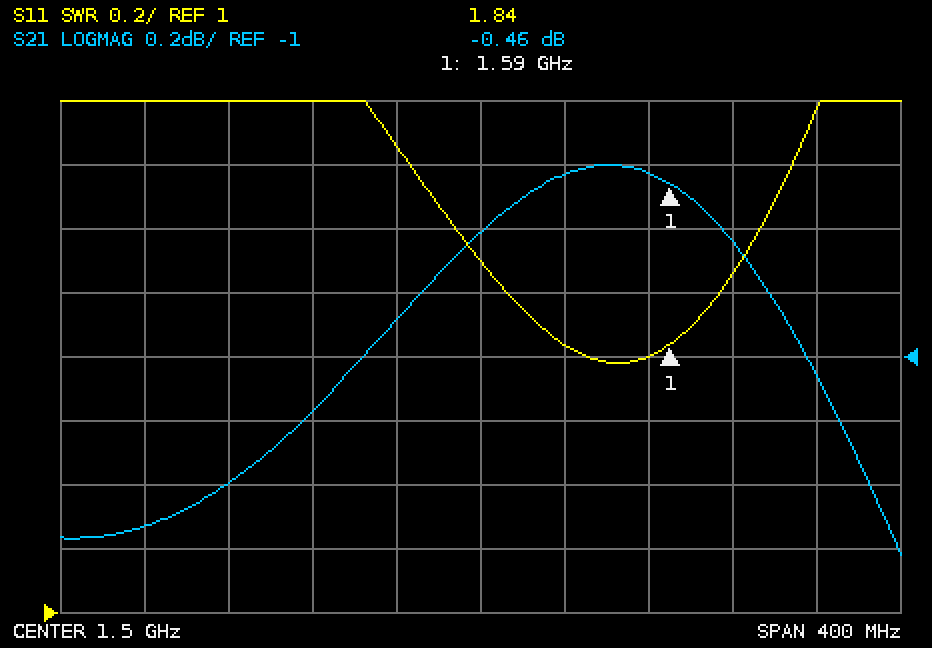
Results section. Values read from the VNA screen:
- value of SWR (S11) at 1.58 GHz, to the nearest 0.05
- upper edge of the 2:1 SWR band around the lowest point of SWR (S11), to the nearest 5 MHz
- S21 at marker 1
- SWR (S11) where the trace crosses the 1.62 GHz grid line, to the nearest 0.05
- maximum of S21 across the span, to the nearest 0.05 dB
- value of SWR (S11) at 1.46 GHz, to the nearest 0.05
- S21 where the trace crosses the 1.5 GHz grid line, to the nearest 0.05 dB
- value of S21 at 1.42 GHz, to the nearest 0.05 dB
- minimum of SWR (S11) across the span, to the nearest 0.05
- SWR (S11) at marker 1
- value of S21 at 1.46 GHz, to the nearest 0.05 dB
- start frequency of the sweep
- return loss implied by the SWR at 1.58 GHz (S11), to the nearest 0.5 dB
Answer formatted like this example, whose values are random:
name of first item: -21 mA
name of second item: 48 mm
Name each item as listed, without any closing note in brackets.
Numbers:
value of SWR (S11) at 1.58 GHz, to the nearest 0.05: 1.80
upper edge of the 2:1 SWR band around the lowest point of SWR (S11), to the nearest 5 MHz: 1.615 GHz
S21 at marker 1: -0.46 dB
SWR (S11) where the trace crosses the 1.62 GHz grid line, to the nearest 0.05: 2.05
maximum of S21 across the span, to the nearest 0.05 dB: -0.40 dB
value of SWR (S11) at 1.46 GHz, to the nearest 0.05: 2.45
S21 where the trace crosses the 1.5 GHz grid line, to the nearest 0.05 dB: -0.60 dB
value of S21 at 1.42 GHz, to the nearest 0.05 dB: -1.15 dB
minimum of SWR (S11) across the span, to the nearest 0.05: 1.80
SWR (S11) at marker 1: 1.84
value of S21 at 1.46 GHz, to the nearest 0.05 dB: -0.90 dB
start frequency of the sweep: 1.3 GHz
return loss implied by the SWR at 1.58 GHz (S11), to the nearest 0.5 dB: 11.0 dB
